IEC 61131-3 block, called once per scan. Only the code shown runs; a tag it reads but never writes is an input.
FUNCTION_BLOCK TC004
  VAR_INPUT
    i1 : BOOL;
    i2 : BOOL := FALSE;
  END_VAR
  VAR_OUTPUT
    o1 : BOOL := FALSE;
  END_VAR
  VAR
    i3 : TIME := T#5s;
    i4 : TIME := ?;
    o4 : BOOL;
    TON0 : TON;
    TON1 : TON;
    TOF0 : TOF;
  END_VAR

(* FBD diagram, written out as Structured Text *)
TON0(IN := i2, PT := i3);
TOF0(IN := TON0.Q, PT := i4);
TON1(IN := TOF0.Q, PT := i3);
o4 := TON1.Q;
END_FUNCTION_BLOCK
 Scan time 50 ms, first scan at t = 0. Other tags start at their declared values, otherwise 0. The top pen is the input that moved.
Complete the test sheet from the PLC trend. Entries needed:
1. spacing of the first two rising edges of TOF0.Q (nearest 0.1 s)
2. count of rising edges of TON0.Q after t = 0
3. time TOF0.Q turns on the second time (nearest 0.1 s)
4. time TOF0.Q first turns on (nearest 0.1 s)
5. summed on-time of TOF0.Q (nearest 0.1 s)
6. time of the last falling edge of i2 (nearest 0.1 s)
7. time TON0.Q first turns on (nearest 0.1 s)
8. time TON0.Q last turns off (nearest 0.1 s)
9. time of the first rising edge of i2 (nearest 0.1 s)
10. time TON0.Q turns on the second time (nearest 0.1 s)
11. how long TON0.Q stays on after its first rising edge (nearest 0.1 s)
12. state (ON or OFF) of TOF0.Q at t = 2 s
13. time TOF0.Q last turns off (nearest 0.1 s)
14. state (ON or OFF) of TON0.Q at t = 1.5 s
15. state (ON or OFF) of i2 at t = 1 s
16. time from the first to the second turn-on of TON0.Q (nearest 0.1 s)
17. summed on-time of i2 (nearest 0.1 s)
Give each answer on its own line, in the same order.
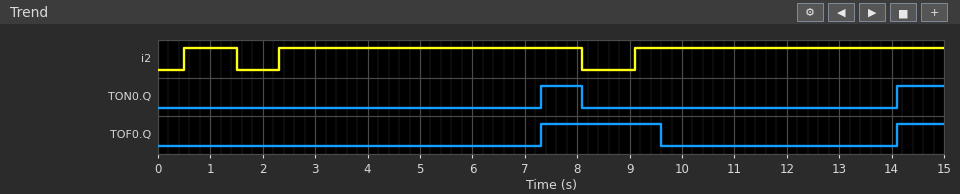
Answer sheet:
6.8 s
2
14.1 s
7.3 s
3.2 s
8.1 s
7.3 s
8.1 s
0.5 s
14.1 s
0.8 s
OFF
9.6 s
OFF
ON
6.8 s
12.7 s
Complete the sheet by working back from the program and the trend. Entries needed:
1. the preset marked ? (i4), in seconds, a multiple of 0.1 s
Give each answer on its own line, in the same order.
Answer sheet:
1.5 s
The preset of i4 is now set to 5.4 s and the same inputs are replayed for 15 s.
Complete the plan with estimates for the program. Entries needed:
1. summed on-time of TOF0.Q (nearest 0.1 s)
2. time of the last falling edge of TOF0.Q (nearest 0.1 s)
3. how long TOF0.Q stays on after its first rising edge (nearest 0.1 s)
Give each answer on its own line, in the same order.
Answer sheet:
7.1 s
13.5 s
6.2 s
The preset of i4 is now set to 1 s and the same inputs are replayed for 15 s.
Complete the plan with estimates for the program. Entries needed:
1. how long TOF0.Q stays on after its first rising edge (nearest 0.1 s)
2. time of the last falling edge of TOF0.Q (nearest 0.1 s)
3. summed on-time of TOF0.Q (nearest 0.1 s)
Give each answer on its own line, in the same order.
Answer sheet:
1.8 s
9.1 s
2.7 s
